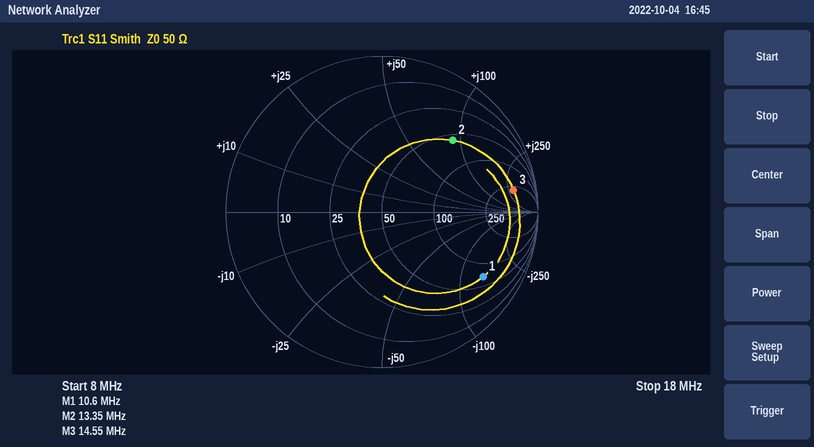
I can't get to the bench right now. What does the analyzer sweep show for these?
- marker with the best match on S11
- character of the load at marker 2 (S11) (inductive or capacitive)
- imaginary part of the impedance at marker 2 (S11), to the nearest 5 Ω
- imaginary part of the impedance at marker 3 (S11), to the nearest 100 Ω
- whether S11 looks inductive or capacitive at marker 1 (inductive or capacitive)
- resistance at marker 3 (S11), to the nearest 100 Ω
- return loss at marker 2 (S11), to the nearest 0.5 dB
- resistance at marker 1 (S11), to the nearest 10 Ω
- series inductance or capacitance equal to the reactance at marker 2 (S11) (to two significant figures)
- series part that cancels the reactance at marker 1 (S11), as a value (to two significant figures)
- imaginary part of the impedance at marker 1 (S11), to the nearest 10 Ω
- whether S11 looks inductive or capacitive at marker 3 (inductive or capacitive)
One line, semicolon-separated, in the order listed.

marker 2; inductive; +90 Ω; +300 Ω; capacitive; 300 Ω; 4.0 dB; 70 Ω; 1.1 µH; 2.1 µH; -140 Ω; inductive
